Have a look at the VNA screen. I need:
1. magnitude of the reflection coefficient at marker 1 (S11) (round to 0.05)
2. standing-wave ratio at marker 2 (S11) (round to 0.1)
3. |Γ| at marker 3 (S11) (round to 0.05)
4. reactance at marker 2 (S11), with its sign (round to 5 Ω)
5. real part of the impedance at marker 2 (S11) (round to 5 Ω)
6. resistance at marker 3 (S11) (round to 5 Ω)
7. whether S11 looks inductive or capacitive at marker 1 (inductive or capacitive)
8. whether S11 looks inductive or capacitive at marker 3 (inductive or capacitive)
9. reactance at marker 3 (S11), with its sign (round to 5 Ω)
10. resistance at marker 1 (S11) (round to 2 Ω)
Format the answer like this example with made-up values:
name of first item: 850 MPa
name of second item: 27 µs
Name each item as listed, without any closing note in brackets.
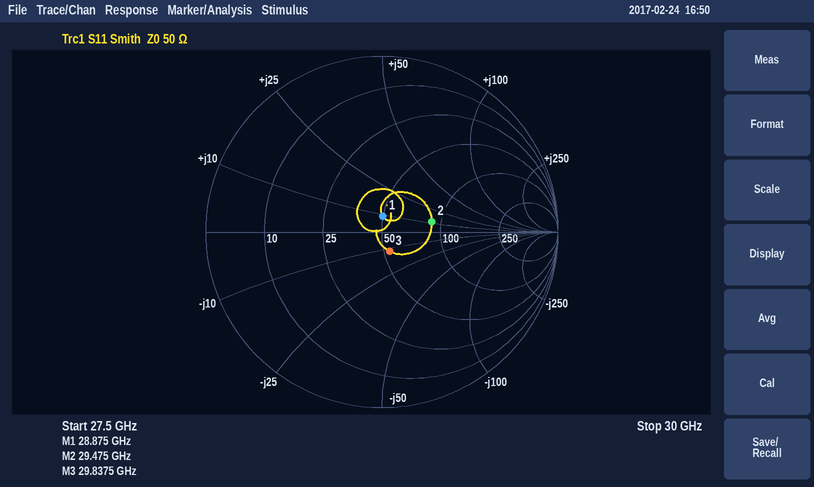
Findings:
magnitude of the reflection coefficient at marker 1 (S11): 0.10
standing-wave ratio at marker 2 (S11): 1.8
|Γ| at marker 3 (S11): 0.10
reactance at marker 2 (S11), with its sign: +10 Ω
real part of the impedance at marker 2 (S11): 90 Ω
resistance at marker 3 (S11): 55 Ω
whether S11 looks inductive or capacitive at marker 1: inductive
whether S11 looks inductive or capacitive at marker 3: capacitive
reactance at marker 3 (S11), with its sign: -10 Ω
resistance at marker 1 (S11): 50 Ω
